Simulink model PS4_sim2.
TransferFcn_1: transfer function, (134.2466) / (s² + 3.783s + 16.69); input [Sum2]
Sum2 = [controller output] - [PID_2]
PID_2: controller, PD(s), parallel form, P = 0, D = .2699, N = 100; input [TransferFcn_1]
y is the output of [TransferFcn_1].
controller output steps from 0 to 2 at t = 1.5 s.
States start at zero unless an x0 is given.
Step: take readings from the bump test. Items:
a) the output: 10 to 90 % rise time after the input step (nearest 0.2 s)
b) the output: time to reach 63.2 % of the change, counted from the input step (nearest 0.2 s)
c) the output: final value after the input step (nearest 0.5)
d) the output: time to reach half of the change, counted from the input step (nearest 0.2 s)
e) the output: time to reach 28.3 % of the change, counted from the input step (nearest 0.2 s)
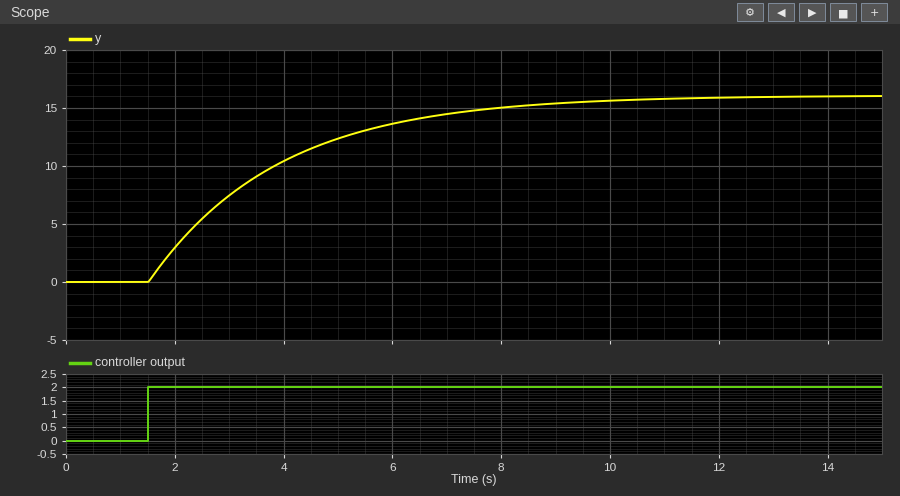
5.2 s
2.4 s
16.0
1.6 s
0.8 s
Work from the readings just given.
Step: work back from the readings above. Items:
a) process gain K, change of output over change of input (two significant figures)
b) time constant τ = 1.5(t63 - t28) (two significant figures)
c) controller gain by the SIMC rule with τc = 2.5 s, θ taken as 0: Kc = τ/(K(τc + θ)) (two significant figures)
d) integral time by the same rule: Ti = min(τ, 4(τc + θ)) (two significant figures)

8.0
2.4 s
0.12
2.4 s
